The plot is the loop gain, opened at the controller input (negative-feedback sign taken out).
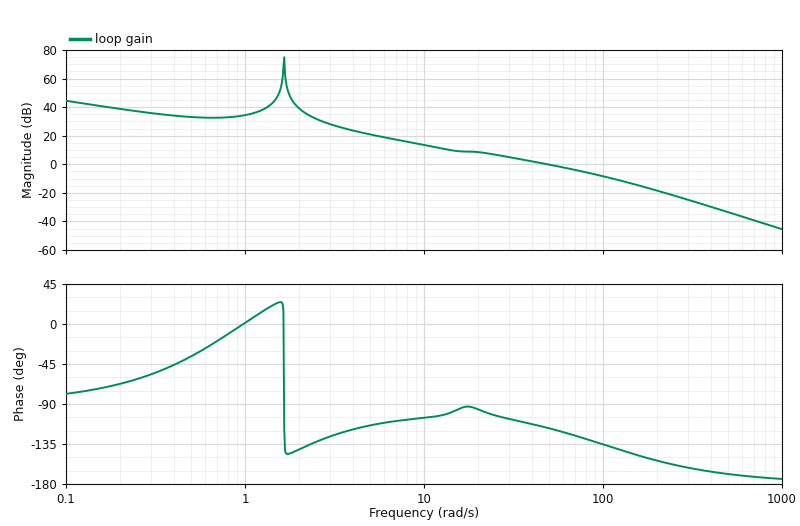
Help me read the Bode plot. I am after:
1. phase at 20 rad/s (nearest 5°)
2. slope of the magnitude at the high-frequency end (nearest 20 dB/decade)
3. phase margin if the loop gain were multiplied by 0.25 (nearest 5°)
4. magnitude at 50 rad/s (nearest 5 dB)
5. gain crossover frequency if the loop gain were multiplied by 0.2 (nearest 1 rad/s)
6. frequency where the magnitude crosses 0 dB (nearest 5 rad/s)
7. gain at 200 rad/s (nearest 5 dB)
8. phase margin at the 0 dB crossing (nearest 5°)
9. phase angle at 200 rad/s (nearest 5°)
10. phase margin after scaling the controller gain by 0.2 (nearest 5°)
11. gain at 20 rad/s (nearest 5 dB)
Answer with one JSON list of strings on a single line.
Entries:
["-95°", "-40 dB/decade", "75°", "0 dB", "10 rad/s", "50 rad/s", "-20 dB", "65°", "-155°", "75°", "10 dB"]
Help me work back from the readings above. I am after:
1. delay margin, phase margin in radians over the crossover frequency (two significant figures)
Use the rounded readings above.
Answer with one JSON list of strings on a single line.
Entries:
["0.023 s"]
